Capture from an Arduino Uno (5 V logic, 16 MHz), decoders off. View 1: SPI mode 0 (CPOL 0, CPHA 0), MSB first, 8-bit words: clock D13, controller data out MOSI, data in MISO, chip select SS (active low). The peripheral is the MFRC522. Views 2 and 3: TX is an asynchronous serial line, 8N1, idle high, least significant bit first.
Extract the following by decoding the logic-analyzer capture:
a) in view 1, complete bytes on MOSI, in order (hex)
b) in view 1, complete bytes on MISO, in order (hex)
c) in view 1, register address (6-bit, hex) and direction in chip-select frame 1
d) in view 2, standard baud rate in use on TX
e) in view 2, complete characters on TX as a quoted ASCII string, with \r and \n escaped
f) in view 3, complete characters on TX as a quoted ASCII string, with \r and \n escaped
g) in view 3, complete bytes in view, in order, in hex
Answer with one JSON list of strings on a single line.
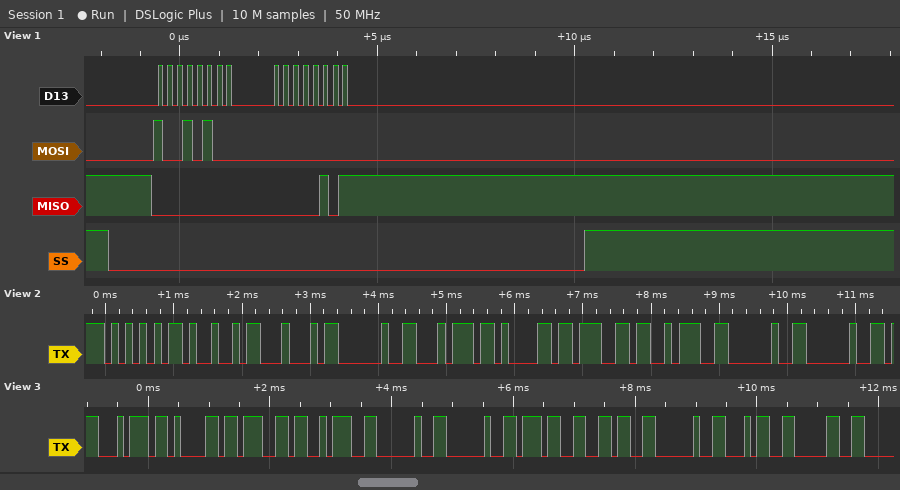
["0x94 0x00", "0x00 0x05", "0x0A read", "9600 baud", "\"UID tag:  \"", "\"tag:  76 40\"", "74 61 67 3A 20 20 37 36 20 34 30"]
